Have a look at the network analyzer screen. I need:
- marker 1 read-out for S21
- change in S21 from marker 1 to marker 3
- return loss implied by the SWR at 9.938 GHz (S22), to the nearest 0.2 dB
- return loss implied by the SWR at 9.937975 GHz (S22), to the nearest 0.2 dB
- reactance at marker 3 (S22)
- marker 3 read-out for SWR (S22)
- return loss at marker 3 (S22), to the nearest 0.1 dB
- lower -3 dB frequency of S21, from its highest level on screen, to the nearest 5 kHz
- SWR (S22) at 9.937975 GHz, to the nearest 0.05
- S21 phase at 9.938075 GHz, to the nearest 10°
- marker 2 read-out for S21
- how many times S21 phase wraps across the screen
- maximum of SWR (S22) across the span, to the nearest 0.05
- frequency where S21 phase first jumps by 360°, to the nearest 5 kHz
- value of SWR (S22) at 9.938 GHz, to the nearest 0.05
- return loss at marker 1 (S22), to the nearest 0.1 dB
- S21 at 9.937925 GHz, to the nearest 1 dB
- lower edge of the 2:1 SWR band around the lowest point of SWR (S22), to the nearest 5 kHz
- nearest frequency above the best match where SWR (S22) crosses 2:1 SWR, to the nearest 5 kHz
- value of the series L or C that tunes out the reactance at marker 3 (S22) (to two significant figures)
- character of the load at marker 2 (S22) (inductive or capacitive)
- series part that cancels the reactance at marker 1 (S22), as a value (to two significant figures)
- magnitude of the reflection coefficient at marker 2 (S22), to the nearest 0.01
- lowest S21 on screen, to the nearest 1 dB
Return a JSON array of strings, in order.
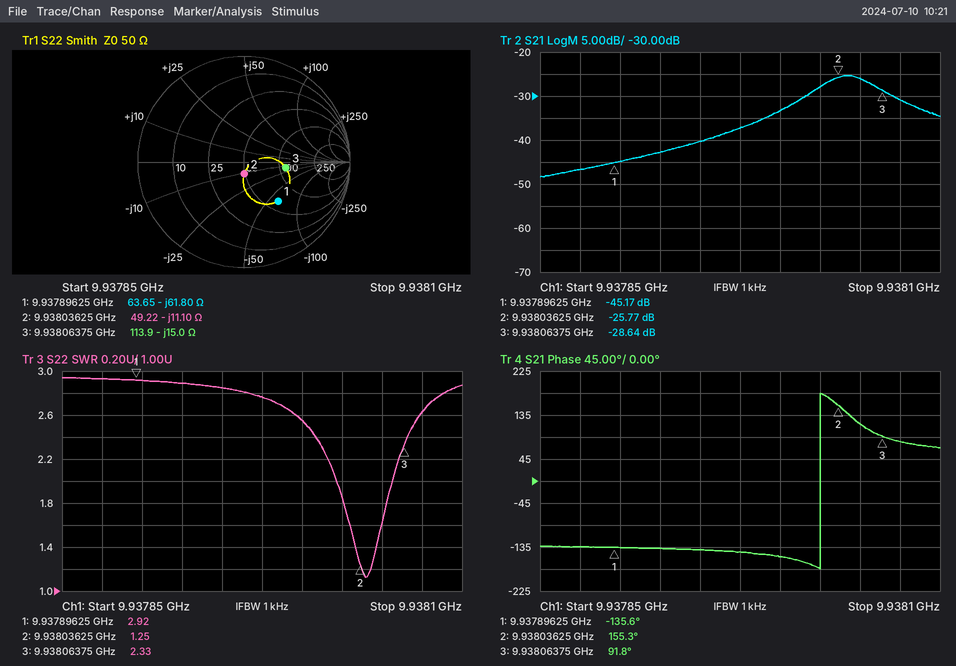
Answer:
["-45.17 dB", "16.53 dB", "7.2 dB", "6.6 dB", "-15.0 Ω", "2.33", "8.0 dB", "9.938025 GHz", "2.75", "80°", "-25.77 dB", "1", "2.95", "9.938025 GHz", "2.55", "6.2 dB", "-43 dB", "9.938020 GHz", "9.938055 GHz", "240 pH", "capacitive", "990 pH", "0.11", "-48 dB"]
